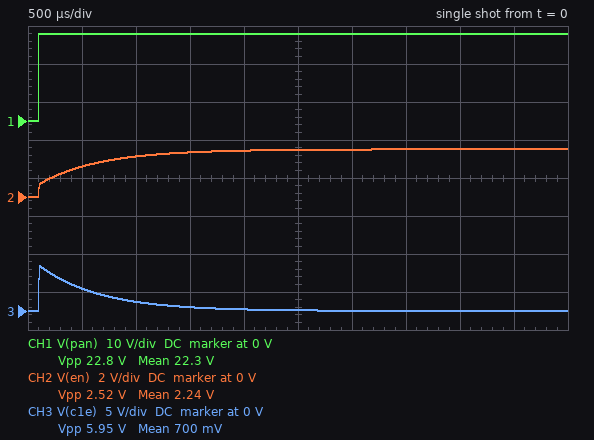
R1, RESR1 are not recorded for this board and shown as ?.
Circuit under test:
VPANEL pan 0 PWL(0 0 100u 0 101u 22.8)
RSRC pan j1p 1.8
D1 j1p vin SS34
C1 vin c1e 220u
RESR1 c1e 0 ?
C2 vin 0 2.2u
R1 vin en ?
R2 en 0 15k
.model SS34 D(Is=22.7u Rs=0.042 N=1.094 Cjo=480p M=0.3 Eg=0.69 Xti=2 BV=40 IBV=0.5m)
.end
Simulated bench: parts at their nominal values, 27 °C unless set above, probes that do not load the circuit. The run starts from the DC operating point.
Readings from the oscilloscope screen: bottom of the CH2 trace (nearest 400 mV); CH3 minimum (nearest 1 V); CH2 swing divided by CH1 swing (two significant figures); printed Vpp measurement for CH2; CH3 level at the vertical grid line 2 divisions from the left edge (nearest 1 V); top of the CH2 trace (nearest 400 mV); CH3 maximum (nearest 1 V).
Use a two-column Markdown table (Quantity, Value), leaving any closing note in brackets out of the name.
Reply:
| Quantity | Value |
|---|---|
| bottom of the CH2 trace | 0 V |
| CH3 minimum | 0 V |
| CH2 swing divided by CH1 swing | 0.11 |
| printed Vpp measurement for CH2 | 2.52 V |
| CH3 level at the vertical grid line 2 divisions from the left edge | 1 V |
| top of the CH2 trace | 2.4 V |
| CH3 maximum | 6 V |
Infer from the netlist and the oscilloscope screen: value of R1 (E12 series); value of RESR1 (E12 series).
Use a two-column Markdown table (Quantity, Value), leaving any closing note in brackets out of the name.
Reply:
| Quantity | Value |
|---|---|
| value of R1 | 120 kΩ |
| value of RESR1 | 0.68 Ω |
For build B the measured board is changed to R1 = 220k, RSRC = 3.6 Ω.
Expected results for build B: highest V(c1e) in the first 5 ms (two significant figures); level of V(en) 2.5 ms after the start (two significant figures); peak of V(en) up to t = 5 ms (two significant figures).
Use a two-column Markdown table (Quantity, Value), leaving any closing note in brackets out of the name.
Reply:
| Quantity | Value |
|---|---|
| highest V(c1e) in the first 5 ms | 3.5 V |
| level of V(en) 2.5 ms after the start | 1.3 V |
| peak of V(en) up to t = 5 ms | 1.4 V |
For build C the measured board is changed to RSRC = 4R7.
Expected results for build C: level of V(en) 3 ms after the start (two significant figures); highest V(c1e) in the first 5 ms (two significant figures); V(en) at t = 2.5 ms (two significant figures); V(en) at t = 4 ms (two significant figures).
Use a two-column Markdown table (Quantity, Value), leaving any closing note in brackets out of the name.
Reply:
| Quantity | Value |
|---|---|
| level of V(en) 3 ms after the start | 2.3 V |
| highest V(c1e) in the first 5 ms | 2.8 V |
| V(en) at t = 2.5 ms | 2.2 V |
| V(en) at t = 4 ms | 2.4 V |
